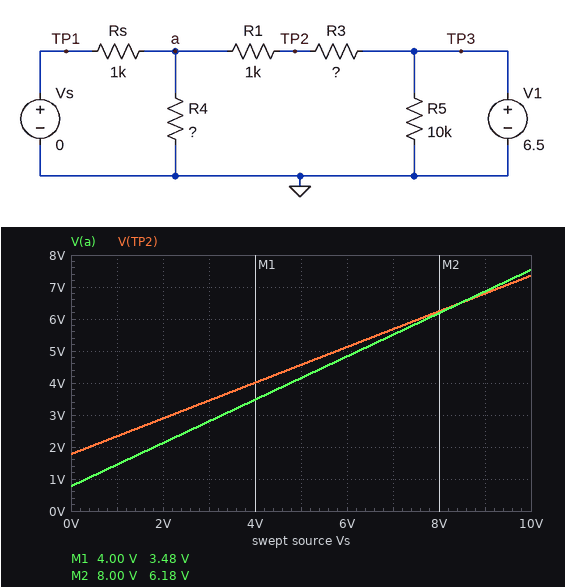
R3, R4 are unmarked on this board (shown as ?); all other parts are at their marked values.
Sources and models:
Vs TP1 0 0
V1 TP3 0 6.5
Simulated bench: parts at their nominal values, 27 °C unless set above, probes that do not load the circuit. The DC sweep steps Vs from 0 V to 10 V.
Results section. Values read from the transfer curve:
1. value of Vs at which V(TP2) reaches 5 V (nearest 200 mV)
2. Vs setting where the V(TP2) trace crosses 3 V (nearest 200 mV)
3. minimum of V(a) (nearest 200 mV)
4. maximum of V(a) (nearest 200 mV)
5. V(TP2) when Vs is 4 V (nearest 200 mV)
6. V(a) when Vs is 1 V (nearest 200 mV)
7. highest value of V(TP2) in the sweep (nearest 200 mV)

5.8 V
2.2 V
800 mV
7.6 V
4.0 V
1.4 V
7.4 V
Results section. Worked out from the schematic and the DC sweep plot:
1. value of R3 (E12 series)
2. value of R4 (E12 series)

4.7 kΩ
3.3 kΩ
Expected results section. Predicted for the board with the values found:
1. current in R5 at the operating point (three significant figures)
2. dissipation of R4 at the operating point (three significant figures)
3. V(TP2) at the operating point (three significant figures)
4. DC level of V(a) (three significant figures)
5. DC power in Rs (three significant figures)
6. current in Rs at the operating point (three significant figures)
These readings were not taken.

650 µA
180 µW
1.78 V
771 mV
595 µW
771 µA
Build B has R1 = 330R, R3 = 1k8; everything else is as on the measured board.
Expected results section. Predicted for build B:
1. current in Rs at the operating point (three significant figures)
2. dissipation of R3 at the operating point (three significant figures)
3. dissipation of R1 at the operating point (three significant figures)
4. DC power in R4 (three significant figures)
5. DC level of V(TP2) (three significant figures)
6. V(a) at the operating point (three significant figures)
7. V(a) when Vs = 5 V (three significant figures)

1.72 mA
9.06 mW
1.66 mW
898 µW
2.46 V
1.72 V
4.54 V
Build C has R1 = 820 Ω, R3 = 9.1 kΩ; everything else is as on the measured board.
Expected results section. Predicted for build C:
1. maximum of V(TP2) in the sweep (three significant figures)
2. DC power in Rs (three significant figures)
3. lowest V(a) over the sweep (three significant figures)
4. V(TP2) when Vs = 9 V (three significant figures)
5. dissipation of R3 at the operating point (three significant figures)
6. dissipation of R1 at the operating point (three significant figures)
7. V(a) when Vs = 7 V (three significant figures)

7.50 V
218 µW
467 mV
6.85 V
3.37 mW
303 µW
5.45 V
